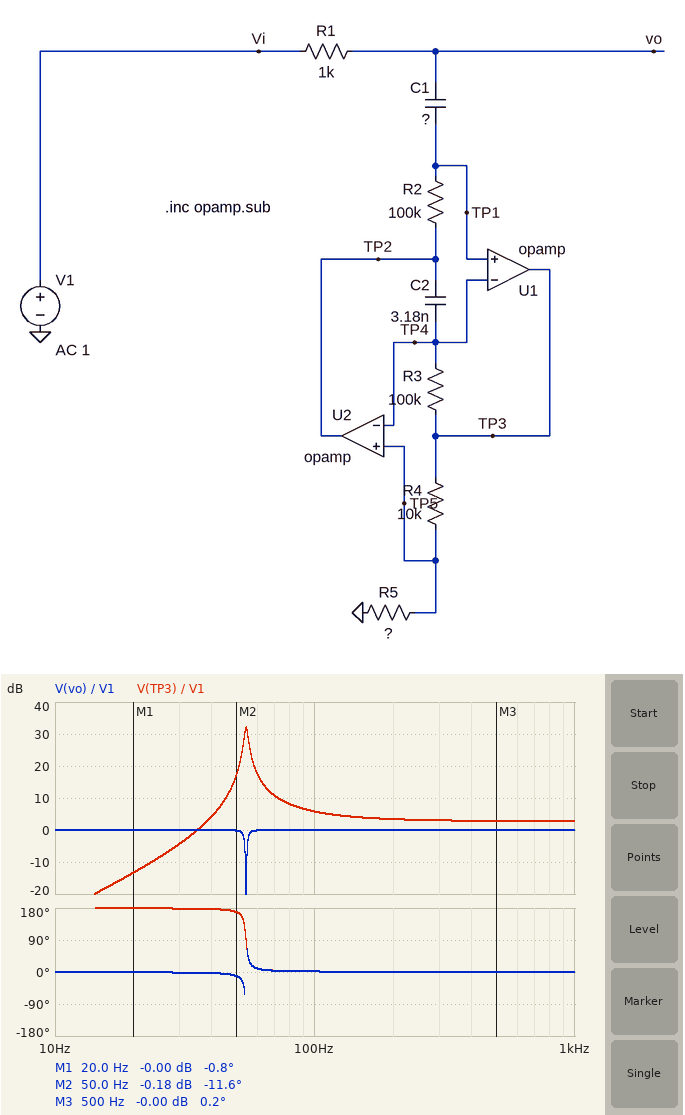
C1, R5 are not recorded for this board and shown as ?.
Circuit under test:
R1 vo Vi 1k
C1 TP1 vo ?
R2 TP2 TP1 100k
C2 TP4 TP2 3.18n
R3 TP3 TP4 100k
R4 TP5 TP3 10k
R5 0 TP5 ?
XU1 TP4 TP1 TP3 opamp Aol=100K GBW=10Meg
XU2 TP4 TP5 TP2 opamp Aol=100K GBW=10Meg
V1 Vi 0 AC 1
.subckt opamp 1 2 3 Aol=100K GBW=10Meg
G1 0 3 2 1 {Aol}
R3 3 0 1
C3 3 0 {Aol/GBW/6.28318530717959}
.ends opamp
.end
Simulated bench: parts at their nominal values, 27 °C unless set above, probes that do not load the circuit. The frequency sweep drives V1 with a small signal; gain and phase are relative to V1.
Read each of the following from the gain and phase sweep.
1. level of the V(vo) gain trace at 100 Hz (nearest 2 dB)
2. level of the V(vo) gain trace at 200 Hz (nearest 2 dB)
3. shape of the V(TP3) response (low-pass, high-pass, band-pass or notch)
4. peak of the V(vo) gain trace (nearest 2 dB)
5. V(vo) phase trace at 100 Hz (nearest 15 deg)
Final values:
0 dB
0 dB
high-pass
0 dB
0 deg
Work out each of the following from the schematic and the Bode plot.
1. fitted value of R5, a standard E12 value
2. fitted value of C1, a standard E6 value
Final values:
27 kΩ
100 nF
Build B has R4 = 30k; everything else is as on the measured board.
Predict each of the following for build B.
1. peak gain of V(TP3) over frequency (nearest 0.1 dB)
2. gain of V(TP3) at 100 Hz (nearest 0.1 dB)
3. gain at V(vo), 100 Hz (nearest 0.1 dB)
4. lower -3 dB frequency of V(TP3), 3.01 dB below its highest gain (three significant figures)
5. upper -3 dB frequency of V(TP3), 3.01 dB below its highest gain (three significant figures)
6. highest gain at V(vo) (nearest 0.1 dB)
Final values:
31.0 dB
24.4 dB
-0.9 dB
91.5 Hz
97.1 Hz
0 dB
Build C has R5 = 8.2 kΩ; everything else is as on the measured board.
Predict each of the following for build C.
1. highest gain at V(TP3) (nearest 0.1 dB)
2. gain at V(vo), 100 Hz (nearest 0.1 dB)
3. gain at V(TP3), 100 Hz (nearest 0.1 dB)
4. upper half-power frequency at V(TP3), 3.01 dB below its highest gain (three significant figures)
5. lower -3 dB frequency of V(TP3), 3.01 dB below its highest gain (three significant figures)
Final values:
31.1 dB
-7.4 dB
30.3 dB
102 Hz
95.7 Hz
